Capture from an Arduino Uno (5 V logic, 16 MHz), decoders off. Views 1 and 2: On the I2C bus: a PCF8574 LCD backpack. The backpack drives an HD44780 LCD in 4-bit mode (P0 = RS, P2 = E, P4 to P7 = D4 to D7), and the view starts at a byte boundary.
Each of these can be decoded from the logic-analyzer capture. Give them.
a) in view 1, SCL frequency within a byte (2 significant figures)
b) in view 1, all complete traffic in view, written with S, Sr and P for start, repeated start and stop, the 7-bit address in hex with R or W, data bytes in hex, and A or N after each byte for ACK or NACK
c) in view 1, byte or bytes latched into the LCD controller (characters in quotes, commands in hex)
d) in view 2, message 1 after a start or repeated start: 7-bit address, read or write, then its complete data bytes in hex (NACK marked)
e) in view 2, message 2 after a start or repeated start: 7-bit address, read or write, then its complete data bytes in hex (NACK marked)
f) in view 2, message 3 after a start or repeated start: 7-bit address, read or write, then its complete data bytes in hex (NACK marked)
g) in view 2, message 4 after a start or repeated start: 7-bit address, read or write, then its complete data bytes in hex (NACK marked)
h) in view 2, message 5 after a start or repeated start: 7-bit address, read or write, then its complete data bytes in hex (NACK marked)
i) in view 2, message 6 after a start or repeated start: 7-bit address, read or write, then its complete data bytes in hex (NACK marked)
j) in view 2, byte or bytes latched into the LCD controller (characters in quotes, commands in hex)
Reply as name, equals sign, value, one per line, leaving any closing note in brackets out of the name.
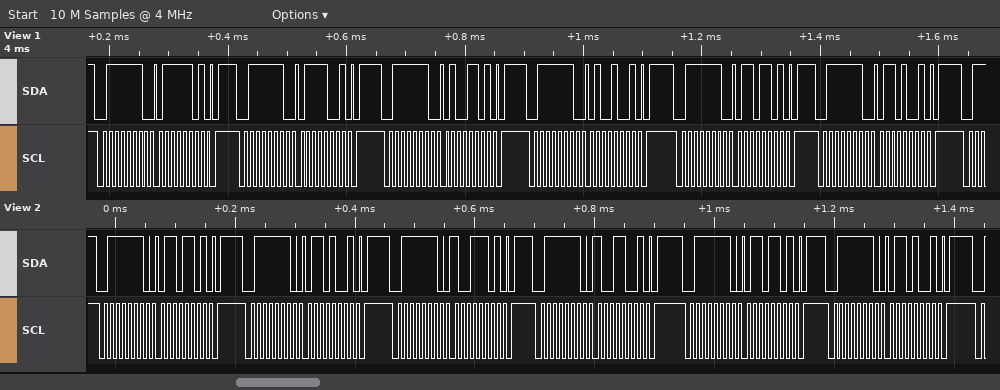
in view 1, SCL frequency within a byte = 100 kHz
in view 1, all complete traffic in view, written with S, Sr and P for start, repeated start and stop, the 7-bit address in hex with R or W, data bytes in hex, and A or N after each byte for ACK or NACK = S 3FW A 7D A P S 3FW A 79 A P S 3FW A 4D A P S 3FW A 49 A P S 3FW A 6D A P S 3FW A 69 A P
in view 1, byte or bytes latched into the LCD controller = 't'
in view 2, message 1 after a start or repeated start: 7-bit address, read or write, then its complete data bytes in hex = 0x3F write: 6D
in view 2, message 2 after a start or repeated start: 7-bit address, read or write, then its complete data bytes in hex = 0x3F write: 69
in view 2, message 3 after a start or repeated start: 7-bit address, read or write, then its complete data bytes in hex = 0x3F write: 9D
in view 2, message 4 after a start or repeated start: 7-bit address, read or write, then its complete data bytes in hex = 0x3F write: 99
in view 2, message 5 after a start or repeated start: 7-bit address, read or write, then its complete data bytes in hex = 0x3F write: 6D
in view 2, message 6 after a start or repeated start: 7-bit address, read or write, then its complete data bytes in hex = 0x3F write: 69
in view 2, byte or bytes latched into the LCD controller = 'i'
